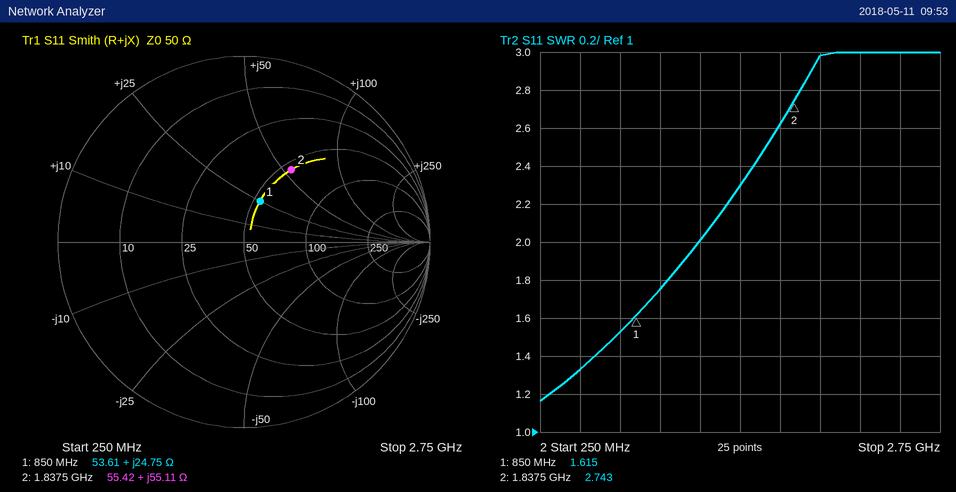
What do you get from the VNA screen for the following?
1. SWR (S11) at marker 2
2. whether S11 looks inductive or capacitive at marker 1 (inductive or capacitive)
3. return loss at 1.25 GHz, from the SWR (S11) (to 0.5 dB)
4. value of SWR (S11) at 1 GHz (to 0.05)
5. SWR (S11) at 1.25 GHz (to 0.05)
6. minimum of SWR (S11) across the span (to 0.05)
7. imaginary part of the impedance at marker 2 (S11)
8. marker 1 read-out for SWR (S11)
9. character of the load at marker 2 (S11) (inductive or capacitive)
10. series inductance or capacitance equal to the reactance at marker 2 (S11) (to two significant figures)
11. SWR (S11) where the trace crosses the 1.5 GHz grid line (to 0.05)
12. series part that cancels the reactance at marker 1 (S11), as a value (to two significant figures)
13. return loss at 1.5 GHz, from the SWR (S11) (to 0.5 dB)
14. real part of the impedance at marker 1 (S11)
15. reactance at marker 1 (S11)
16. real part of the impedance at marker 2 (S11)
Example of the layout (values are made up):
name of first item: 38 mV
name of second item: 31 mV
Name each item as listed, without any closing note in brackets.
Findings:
SWR (S11) at marker 2: 2.743
whether S11 looks inductive or capacitive at marker 1: inductive
return loss at 1.25 GHz, from the SWR (S11): 9.5 dB
value of SWR (S11) at 1 GHz: 1.75
SWR (S11) at 1.25 GHz: 2.00
minimum of SWR (S11) across the span: 1.15
imaginary part of the impedance at marker 2: +55.11 Ω
marker 1 read-out for SWR: 1.615
character of the load at marker 2 (S11): inductive
series inductance or capacitance equal to the reactance at marker 2 (S11): 4.8 nH
SWR (S11) where the trace crosses the 1.5 GHz grid line: 2.30
series part that cancels the reactance at marker 1 (S11), as a value: 7.6 pF
return loss at 1.5 GHz, from the SWR (S11): 8.0 dB
real part of the impedance at marker 1: 53.61 Ω
reactance at marker 1: +24.75 Ω
real part of the impedance at marker 2: 55.42 Ω
